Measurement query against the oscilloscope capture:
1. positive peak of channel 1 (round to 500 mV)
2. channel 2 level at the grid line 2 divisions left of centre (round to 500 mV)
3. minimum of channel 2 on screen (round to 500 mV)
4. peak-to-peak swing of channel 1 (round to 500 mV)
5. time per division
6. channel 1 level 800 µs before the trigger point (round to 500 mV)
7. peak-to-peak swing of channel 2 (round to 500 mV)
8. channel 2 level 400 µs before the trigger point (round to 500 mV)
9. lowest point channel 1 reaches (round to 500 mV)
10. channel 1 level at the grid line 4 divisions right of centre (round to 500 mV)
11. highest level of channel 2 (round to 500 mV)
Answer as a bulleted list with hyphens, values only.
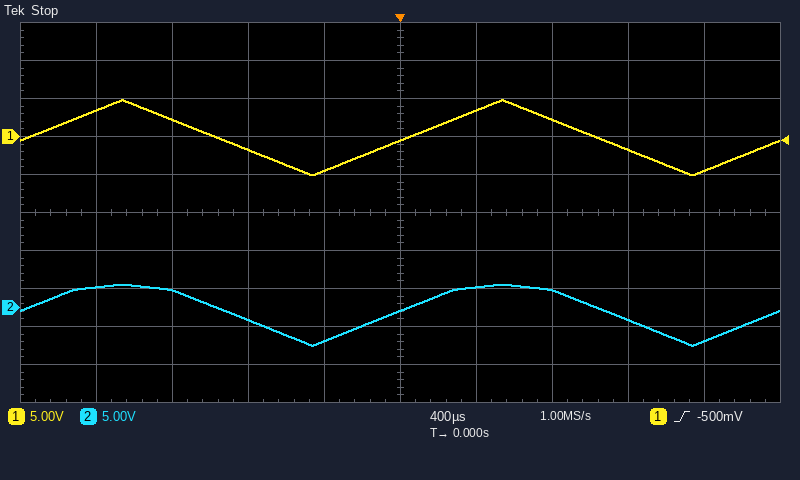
- 5.0 V
- -1.5 V
- -5.0 V
- 10.0 V
- 400 µs
- -1.5 V
- 8.0 V
- -4.5 V
- -5.0 V
- -4.5 V
- 3.0 V
